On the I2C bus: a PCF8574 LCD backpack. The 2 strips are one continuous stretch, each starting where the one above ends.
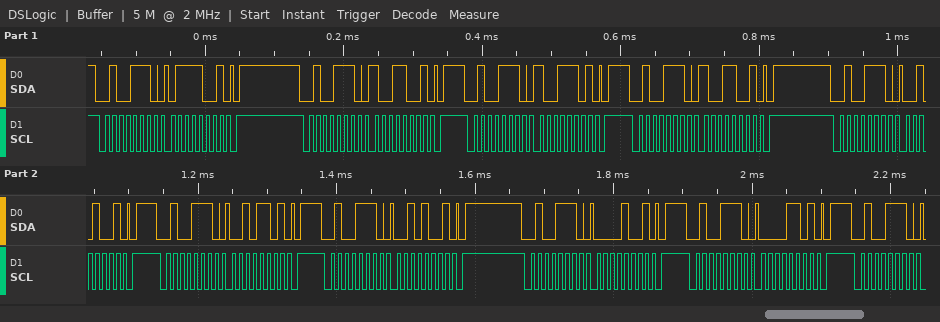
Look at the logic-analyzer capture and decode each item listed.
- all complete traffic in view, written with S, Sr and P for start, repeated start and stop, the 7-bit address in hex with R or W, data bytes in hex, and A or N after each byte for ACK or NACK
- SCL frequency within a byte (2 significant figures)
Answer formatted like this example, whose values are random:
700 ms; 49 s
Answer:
S 27W A 79 A P S 27W A 99 A P S 27W A 9D A P S 27W A 99 A P S 27W A 29 A P S 27W A 2D A P S 27W A 29 A P S 27W A 09 A P S 27W A 0D A P S 27W A; 100 kHz
